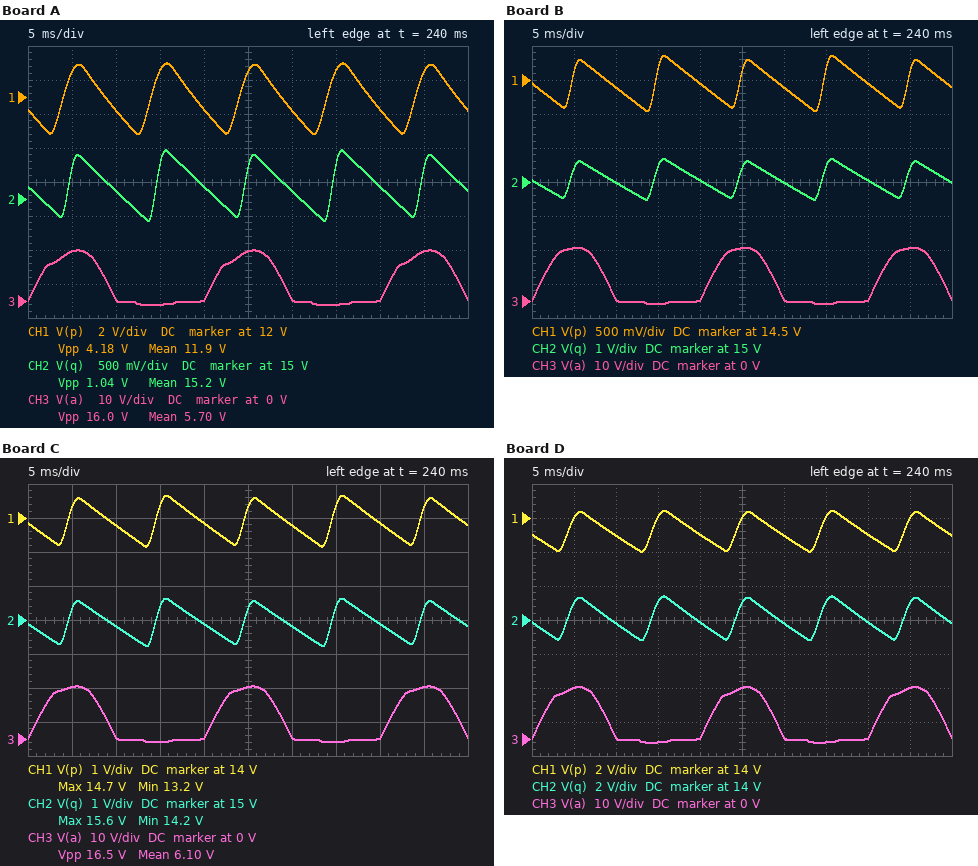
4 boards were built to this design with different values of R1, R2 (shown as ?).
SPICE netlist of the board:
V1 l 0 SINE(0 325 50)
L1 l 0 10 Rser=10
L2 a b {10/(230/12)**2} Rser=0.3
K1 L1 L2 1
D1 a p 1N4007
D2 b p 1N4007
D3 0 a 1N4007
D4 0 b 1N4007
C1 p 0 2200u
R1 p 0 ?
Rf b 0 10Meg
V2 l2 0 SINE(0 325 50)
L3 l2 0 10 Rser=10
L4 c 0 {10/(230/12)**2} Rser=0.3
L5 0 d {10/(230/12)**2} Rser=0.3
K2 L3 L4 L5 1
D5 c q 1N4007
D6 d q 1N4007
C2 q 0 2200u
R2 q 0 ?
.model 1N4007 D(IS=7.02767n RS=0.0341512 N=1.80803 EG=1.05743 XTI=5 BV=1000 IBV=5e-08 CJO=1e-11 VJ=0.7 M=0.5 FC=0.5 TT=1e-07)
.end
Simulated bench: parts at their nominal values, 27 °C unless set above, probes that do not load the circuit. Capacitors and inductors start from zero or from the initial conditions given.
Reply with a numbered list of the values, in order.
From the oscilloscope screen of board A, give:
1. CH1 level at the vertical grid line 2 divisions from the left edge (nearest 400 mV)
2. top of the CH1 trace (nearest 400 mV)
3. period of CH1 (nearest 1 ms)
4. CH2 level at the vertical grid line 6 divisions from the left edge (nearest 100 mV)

1. 11.2 V
2. 14.0 V
3. 10 ms
4. 15.1 V
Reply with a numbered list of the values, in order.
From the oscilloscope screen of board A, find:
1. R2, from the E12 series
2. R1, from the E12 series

1. 56 Ω
2. 8.2 Ω
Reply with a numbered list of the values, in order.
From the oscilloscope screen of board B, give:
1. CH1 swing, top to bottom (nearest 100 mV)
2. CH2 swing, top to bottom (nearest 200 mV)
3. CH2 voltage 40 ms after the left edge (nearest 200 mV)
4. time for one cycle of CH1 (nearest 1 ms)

1. 800 mV
2. 1.2 V
3. 15.0 V
4. 10 ms
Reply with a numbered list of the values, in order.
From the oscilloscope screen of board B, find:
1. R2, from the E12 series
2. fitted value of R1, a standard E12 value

1. 47 Ω
2. 68 Ω
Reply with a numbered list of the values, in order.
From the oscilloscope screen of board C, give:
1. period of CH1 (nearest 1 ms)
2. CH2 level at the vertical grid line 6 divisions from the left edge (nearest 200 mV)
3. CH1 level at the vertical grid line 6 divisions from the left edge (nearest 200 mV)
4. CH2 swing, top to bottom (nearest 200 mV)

1. 10 ms
2. 14.8 V
3. 13.8 V
4. 1.4 V
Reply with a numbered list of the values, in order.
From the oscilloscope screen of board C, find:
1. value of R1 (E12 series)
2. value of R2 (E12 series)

1. 33 Ω
2. 39 Ω
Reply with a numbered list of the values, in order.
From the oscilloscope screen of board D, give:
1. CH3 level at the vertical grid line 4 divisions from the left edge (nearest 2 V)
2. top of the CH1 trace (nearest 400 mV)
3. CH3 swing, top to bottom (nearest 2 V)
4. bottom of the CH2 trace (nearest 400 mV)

1. 0 V
2. 14.4 V
3. 16 V
4. 12.8 V
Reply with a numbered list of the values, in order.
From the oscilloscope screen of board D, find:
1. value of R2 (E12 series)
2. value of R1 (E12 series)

1. 18 Ω
2. 18 Ω
